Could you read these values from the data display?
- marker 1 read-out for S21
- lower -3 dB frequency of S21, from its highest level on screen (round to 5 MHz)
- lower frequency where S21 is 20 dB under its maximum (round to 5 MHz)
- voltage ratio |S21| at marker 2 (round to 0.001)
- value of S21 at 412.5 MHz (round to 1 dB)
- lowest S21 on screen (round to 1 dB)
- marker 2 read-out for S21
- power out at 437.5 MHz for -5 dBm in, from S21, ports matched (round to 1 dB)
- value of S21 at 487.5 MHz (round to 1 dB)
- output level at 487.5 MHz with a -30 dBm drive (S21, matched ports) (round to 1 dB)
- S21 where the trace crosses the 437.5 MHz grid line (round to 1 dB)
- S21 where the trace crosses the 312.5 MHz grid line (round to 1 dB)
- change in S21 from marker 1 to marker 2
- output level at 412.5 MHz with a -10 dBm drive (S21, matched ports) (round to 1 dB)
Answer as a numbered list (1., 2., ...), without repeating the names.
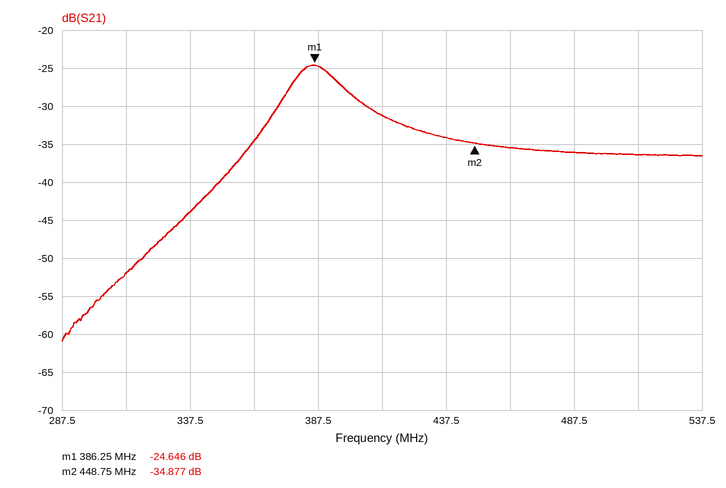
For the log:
1. -24.646 dB
2. 375 MHz
3. 335 MHz
4. 0.018
5. -31 dB
6. -61 dB
7. -34.877 dB
8. -39 dBm
9. -36 dB
10. -66 dBm
11. -34 dB
12. -52 dB
13. -10.231 dB
14. -41 dBm
